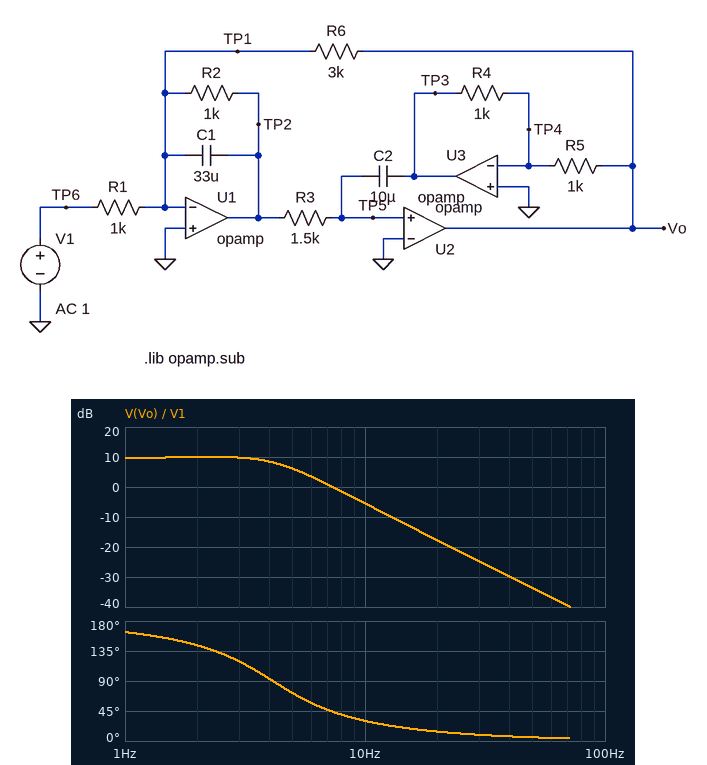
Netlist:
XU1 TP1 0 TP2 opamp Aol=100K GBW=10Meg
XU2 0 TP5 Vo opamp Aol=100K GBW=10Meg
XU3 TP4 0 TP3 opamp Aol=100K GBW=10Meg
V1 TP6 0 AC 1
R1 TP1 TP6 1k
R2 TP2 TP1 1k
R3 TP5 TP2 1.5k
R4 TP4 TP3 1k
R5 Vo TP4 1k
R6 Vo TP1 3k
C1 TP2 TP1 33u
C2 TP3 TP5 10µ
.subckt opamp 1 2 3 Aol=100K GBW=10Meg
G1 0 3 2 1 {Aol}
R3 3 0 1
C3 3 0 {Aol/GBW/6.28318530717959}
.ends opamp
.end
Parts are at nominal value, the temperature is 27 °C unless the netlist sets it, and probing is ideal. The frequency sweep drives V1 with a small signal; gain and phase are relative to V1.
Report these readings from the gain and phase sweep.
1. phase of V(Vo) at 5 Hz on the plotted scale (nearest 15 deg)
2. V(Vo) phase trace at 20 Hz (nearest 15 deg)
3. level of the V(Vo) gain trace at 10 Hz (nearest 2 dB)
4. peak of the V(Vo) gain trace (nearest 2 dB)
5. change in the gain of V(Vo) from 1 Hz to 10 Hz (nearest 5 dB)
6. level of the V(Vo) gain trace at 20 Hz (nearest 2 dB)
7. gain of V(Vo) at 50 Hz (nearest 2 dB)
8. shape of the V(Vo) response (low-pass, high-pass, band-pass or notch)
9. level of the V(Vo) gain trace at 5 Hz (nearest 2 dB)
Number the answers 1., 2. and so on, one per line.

1. 75 deg
2. 15 deg
3. -6 dB
4. 10 dB
5. -15 dB
6. -18 dB
7. -34 dB
8. low-pass
9. 6 dB
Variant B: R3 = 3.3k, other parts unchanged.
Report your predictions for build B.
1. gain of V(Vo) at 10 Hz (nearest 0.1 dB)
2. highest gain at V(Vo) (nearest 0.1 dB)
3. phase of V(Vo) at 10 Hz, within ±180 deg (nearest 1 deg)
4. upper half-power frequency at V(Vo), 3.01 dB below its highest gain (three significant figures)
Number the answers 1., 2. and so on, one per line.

1. -13.0 dB
2. 9.5 dB
3. 28 deg
4. 2.19 Hz
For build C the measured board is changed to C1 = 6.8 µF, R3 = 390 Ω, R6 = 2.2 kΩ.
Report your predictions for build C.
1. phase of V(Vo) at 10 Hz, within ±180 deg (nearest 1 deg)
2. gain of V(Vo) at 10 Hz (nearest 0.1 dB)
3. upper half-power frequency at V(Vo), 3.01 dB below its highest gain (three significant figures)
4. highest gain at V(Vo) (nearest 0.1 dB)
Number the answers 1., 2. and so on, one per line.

1. 145 deg
2. 7.4 dB
3. 23.7 Hz
4. 7.5 dB
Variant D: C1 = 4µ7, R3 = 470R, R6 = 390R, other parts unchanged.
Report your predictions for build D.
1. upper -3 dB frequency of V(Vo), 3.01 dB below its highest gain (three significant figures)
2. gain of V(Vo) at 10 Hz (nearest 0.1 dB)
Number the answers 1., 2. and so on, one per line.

1. 64.1 Hz
2. -7.9 dB
